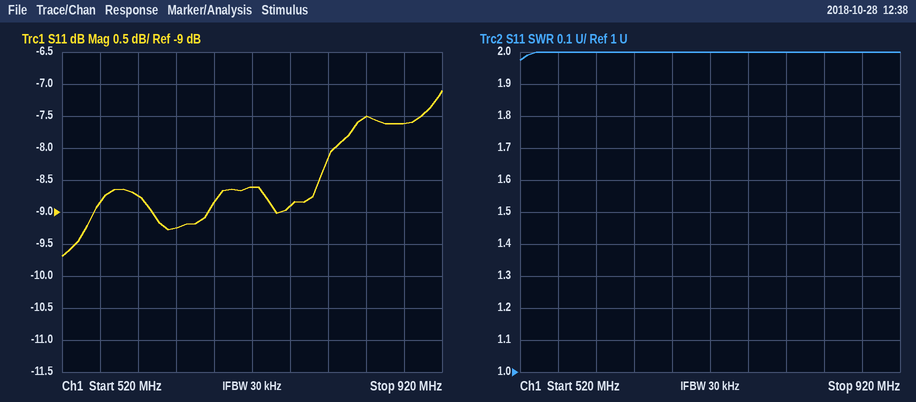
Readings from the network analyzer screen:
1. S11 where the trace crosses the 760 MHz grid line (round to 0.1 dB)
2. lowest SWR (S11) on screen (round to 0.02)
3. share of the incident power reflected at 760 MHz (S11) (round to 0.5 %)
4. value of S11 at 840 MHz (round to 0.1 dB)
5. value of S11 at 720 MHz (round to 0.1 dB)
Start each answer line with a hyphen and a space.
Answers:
- -8.9 dB
- 1.98
- 13.0 %
- -7.5 dB
- -8.6 dB
